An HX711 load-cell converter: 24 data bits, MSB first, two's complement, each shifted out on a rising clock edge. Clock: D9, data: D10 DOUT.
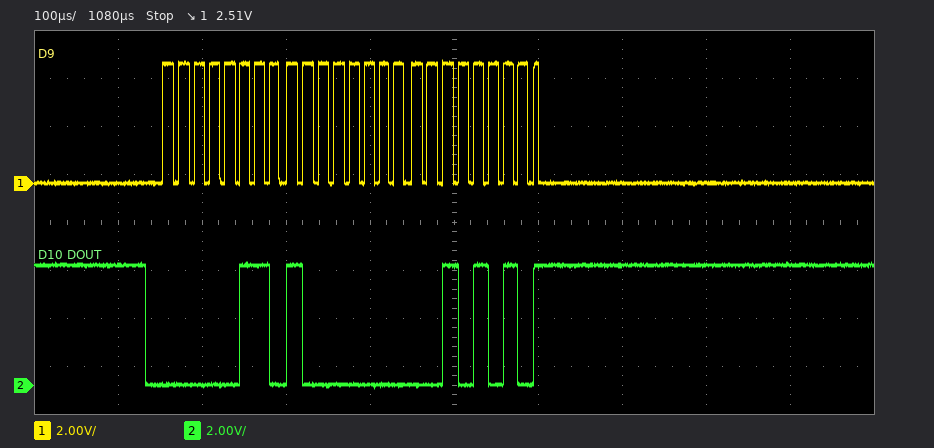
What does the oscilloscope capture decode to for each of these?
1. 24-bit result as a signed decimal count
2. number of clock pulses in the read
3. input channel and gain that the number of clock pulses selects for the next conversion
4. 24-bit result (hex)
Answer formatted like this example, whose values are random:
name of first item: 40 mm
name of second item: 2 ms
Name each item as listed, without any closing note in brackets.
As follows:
24-bit result as a signed decimal count: 426026
number of clock pulses in the read: 25
input channel and gain that the number of clock pulses selects for the next conversion: channel A, gain 128
24-bit result: 0x06802A
